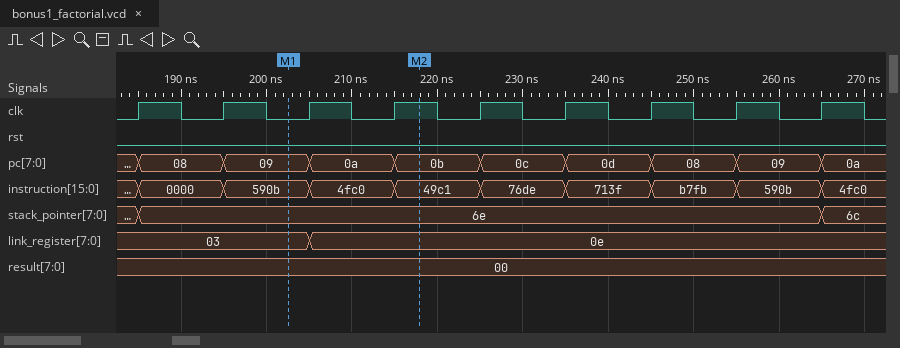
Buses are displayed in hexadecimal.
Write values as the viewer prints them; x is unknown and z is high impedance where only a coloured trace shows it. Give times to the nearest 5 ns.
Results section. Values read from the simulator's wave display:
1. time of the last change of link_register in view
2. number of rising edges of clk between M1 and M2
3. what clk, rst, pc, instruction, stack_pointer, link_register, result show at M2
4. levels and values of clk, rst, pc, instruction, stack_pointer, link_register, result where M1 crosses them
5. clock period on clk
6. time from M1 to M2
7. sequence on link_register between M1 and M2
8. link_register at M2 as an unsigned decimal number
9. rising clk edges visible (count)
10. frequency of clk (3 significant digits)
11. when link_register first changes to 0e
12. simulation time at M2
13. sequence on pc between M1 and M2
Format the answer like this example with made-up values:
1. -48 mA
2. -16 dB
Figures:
1. 205 ns
2. 2
3. clk=1, rst=0, pc=0b, instruction=49c1, stack_pointer=6e, link_register=0e, result=00
4. clk=0, rst=0, pc=09, instruction=590b, stack_pointer=6e, link_register=03, result=00
5. 10 ns
6. 15 ns
7. 03, 0e
8. 14
9. 9
10. 100 MHz
11. 205 ns
12. 220 ns
13. 09, 0a, 0b
